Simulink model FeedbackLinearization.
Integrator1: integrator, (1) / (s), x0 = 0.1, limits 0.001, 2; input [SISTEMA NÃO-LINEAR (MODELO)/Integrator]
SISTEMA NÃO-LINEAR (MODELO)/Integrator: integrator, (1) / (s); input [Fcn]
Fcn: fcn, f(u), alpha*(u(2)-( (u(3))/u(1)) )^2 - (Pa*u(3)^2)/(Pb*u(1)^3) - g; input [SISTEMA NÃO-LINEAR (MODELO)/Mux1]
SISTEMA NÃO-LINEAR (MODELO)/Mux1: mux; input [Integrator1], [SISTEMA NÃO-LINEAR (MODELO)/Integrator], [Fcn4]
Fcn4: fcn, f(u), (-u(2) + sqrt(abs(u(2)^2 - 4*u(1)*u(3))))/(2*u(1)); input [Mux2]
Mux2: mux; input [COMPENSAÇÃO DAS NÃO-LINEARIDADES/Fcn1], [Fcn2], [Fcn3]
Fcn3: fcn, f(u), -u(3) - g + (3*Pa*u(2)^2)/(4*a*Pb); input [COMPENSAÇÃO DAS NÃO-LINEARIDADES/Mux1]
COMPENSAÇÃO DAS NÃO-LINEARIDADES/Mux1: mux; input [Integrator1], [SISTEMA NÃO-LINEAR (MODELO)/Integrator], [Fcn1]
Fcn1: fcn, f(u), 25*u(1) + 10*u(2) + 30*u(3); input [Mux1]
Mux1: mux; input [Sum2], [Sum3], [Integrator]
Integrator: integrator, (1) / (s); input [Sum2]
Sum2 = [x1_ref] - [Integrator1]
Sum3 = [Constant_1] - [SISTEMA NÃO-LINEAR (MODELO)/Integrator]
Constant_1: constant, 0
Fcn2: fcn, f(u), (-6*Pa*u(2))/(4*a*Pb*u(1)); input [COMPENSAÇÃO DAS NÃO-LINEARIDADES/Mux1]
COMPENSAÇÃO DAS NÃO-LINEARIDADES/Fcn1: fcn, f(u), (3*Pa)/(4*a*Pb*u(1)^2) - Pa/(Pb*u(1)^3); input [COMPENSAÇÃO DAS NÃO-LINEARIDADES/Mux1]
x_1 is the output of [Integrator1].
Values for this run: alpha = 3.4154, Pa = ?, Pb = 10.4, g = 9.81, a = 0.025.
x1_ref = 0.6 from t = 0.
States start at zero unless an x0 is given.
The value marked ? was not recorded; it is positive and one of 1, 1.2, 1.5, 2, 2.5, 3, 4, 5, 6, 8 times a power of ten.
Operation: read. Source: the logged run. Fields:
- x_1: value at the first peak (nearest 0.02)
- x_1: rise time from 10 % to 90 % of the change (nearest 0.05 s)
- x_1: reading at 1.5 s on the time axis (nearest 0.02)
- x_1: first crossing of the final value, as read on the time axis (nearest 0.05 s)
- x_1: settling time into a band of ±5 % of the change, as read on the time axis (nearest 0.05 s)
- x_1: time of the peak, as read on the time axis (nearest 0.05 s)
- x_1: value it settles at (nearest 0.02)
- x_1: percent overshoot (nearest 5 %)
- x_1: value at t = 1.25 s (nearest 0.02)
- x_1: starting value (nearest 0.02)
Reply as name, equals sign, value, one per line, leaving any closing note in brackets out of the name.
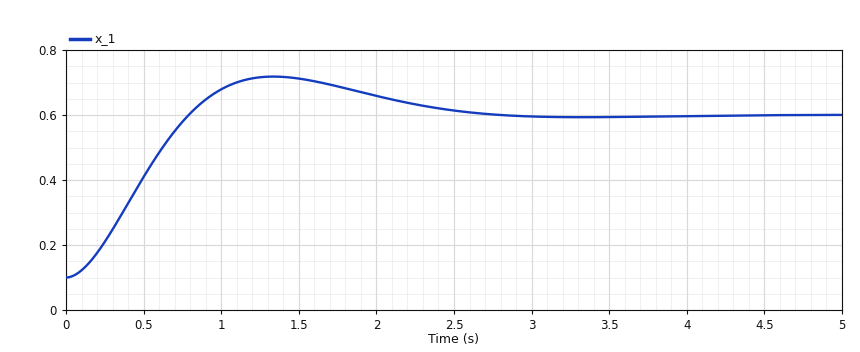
x_1: value at the first peak = 0.72
x_1: rise time from 10 % to 90 % of the change = 0.55 s
x_1: reading at 1.5 s on the time axis = 0.72
x_1: first crossing of the final value, as read on the time axis = 0.80 s
x_1: settling time into a band of ±5 % of the change, as read on the time axis = 2.35 s
x_1: time of the peak, as read on the time axis = 1.35 s
x_1: value it settles at = 0.60
x_1: percent overshoot = 25 %
x_1: value at t = 1.25 s = 0.72
x_1: starting value = 0.10
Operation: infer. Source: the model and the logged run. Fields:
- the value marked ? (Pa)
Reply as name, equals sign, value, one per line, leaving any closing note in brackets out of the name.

the value marked ? = 1.5
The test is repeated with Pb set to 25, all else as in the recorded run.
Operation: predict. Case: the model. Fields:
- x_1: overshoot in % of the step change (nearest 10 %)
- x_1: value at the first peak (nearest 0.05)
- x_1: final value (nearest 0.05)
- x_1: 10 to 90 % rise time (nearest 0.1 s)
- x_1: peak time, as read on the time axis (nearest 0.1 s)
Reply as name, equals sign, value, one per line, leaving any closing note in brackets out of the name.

x_1: overshoot in % of the step change = 40 %
x_1: value at the first peak = 0.80
x_1: final value = 0.60
x_1: 10 to 90 % rise time = 0.3 s
x_1: peak time, as read on the time axis = 1.0 s
